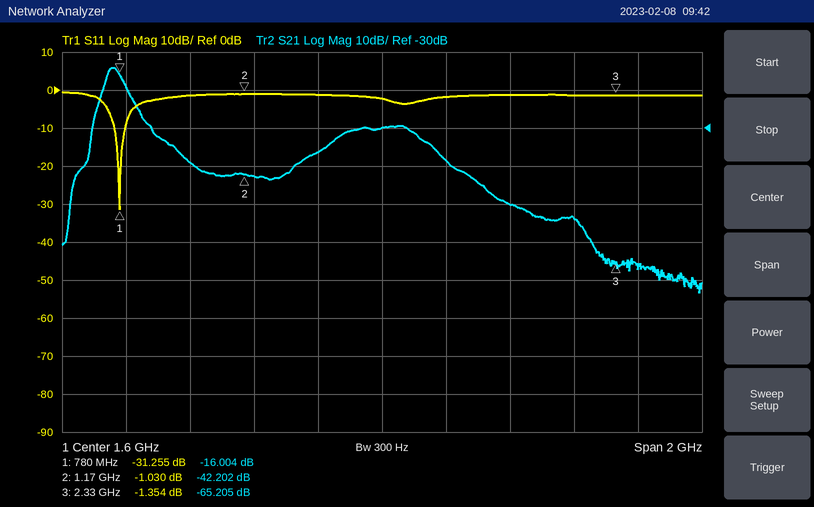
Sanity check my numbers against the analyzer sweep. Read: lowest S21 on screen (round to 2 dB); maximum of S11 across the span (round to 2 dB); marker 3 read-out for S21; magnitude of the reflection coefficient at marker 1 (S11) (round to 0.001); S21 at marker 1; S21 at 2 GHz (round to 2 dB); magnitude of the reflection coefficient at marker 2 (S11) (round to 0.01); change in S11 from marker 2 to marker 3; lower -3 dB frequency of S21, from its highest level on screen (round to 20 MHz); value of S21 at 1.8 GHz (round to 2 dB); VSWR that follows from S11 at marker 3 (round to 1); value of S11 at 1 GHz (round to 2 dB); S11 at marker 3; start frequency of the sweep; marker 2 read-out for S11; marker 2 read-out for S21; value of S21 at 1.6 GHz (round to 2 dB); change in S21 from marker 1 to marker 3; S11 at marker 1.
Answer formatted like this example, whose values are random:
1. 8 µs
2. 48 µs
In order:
1. -74 dB
2. 0 dB
3. -65.205 dB
4. 0.027
5. -16.004 dB
6. -50 dB
7. 0.89
8. -0.324 dB
9. 740 MHz
10. -38 dB
11. 13
12. -2 dB
13. -1.354 dB
14. 600 MHz
15. -1.030 dB
16. -42.202 dB
17. -30 dB
18. -49.201 dB
19. -31.255 dB
